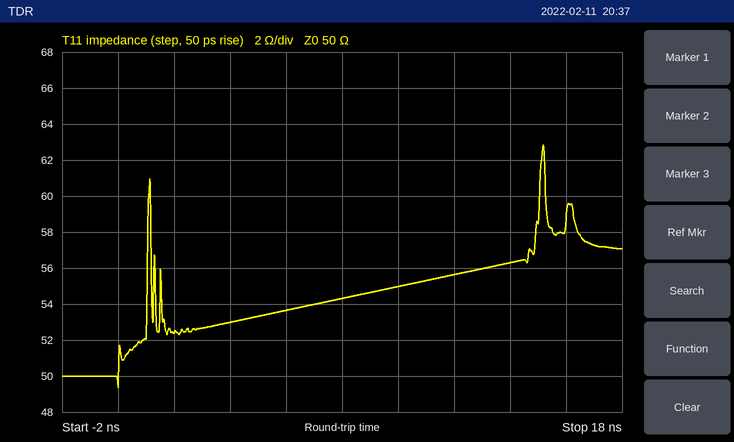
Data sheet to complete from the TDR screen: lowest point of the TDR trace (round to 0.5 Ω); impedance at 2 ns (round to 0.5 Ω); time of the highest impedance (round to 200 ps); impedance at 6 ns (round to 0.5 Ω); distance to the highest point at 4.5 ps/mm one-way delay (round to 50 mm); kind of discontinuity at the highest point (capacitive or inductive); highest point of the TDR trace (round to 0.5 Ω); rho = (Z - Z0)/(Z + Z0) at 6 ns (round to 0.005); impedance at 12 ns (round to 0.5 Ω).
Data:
49.5 Ω
52.5 Ω
15.2 ns
53.5 Ω
1.70 m
inductive
63.0 Ω
+0.035
55.5 Ω
